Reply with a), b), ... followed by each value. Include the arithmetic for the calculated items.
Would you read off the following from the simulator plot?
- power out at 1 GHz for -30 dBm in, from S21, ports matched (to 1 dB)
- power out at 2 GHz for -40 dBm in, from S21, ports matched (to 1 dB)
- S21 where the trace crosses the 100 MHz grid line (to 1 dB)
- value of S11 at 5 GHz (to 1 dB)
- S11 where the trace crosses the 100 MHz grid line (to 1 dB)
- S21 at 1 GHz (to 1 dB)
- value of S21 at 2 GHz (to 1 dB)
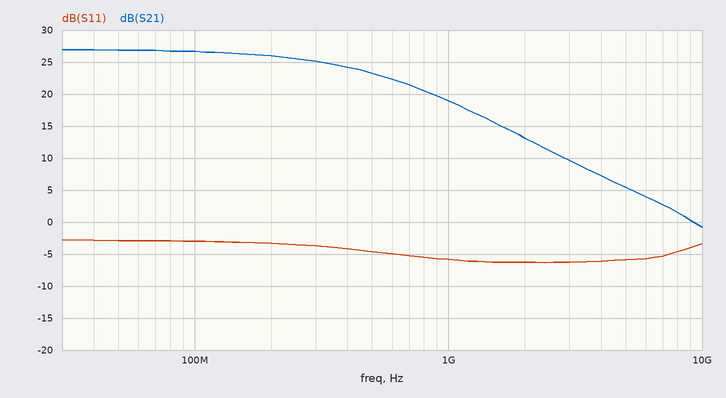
a) -30 dBm + (19 dB) = -11 dBm
b) -40 dBm + (13 dB) = -27 dBm
c) 27 dB
d) -6 dB
e) -3 dB
f) 19 dB
g) 13 dB
